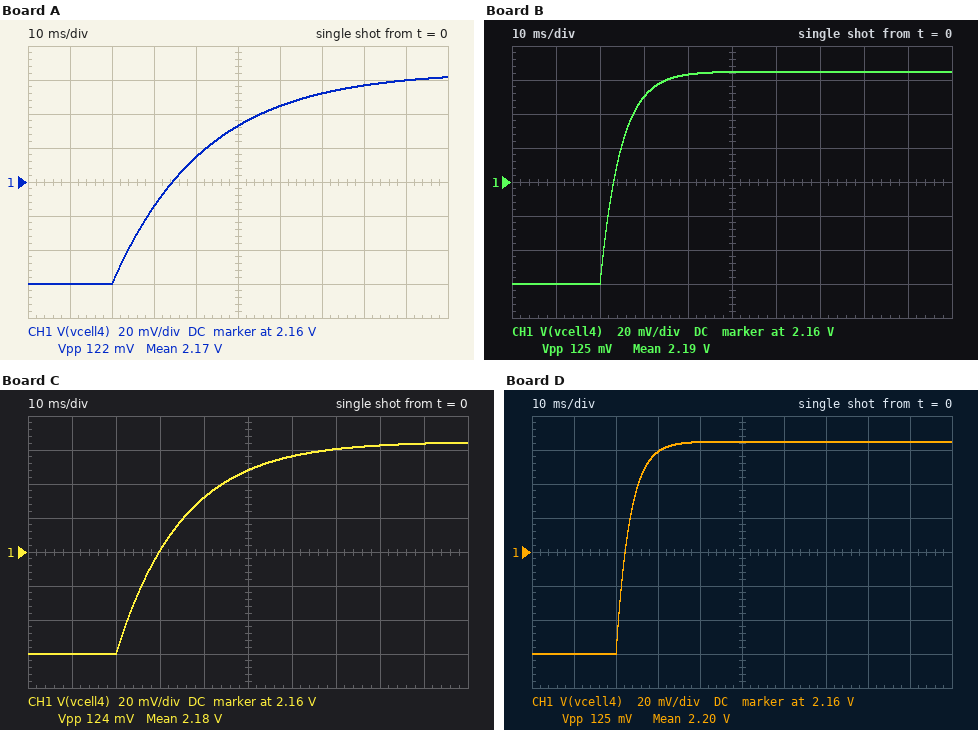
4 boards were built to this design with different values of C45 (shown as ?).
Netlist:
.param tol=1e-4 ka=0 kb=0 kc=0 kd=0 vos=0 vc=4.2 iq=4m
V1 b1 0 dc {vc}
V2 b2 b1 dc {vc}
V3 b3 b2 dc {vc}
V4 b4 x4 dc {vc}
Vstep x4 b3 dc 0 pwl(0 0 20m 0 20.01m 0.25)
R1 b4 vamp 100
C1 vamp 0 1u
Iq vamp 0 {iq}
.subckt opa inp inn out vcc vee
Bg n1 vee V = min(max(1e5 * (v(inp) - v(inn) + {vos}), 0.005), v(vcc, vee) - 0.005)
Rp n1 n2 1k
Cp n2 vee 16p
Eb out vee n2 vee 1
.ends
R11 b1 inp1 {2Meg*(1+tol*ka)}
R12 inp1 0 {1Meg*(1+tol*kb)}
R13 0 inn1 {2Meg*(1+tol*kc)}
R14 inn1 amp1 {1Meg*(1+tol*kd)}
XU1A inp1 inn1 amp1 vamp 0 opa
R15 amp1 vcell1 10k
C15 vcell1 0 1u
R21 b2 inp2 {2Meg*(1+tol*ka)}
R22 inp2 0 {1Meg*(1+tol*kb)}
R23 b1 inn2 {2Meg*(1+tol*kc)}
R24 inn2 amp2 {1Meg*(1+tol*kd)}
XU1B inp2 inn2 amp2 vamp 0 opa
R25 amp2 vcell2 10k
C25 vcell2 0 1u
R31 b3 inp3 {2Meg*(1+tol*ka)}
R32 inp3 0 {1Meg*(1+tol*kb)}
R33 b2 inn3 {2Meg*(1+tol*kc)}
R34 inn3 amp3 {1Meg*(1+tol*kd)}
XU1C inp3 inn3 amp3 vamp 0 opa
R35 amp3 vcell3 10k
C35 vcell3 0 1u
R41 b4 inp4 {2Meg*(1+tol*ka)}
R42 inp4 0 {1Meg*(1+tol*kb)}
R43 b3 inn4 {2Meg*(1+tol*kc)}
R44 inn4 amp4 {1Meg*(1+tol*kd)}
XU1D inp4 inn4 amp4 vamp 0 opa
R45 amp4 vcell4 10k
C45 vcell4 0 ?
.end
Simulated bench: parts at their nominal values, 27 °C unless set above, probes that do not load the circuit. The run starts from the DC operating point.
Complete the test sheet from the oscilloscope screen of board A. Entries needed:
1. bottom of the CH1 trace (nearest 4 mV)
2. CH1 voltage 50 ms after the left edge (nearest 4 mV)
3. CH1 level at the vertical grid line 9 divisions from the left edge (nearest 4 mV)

2.100 V
2.192 V
2.220 V
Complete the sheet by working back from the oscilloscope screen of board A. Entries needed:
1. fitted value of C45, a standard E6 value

2.2 µF
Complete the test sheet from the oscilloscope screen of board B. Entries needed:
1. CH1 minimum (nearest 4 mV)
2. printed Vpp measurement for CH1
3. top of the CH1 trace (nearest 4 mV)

2.100 V
125 mV
2.224 V
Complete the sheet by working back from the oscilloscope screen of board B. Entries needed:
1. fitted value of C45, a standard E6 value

470 nF
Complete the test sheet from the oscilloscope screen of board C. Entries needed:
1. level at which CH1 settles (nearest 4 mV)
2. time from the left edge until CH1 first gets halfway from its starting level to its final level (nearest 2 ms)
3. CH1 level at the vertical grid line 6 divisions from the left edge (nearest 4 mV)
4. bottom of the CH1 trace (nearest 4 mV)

2.224 V
30 ms
2.216 V
2.100 V
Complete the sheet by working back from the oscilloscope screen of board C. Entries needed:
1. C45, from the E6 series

1.5 µF
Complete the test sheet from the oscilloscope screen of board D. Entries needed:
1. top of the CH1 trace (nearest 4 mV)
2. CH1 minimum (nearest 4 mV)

2.224 V
2.100 V
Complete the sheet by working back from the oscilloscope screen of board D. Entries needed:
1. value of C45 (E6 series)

330 nF
